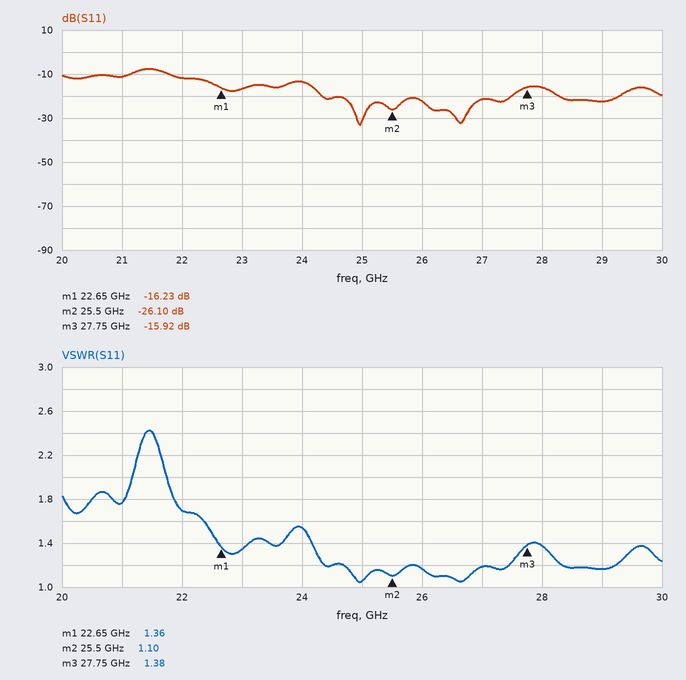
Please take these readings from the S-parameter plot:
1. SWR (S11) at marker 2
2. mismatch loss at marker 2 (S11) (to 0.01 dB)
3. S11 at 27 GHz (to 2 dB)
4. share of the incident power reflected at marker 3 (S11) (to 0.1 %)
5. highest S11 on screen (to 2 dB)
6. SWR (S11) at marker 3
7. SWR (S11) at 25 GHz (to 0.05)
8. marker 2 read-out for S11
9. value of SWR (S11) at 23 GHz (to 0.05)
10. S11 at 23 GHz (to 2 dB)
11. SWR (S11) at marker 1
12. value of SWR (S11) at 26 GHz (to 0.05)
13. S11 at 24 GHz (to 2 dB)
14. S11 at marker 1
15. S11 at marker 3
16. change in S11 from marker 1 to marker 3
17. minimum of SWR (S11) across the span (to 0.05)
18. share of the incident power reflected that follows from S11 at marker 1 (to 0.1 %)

1.10
0.01 dB
-22 dB
2.6 %
-8 dB
1.38
1.05
-26.10 dB
1.35
-16 dB
1.36
1.15
-14 dB
-16.23 dB
-15.92 dB
0.31 dB
1.05
2.4 %
